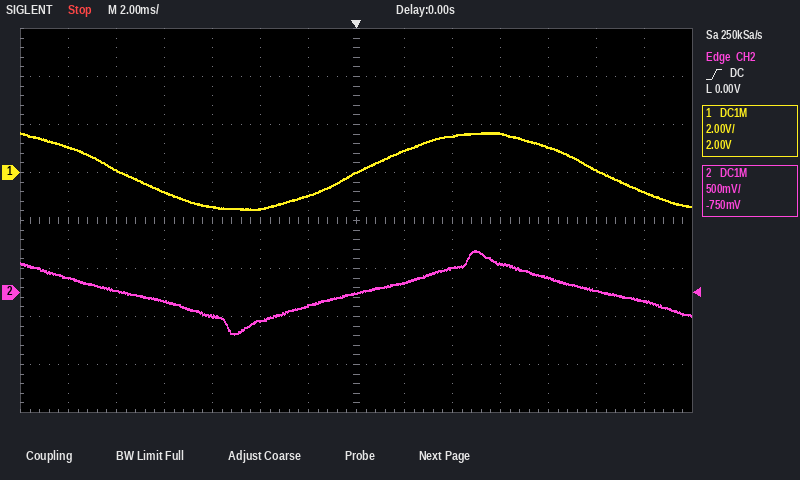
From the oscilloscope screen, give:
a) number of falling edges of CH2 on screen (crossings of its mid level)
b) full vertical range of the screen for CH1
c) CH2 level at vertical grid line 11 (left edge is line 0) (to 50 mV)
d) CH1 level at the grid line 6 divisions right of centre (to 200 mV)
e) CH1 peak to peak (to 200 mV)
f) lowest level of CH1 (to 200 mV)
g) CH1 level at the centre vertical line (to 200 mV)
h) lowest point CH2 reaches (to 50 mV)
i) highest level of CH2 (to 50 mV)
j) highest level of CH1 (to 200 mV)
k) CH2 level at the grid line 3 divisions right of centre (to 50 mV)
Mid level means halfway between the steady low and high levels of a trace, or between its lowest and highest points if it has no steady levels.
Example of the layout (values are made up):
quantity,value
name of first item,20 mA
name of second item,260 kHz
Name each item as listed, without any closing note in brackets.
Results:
quantity,value
number of falling edges of CH2 on screen,2
full vertical range of the screen for CH1,16 V
CH2 level at vertical grid line 11 (left edge is line 0),150 mV
CH1 level at the grid line 6 divisions right of centre,-800 mV
CH1 peak to peak,3.2 V
lowest level of CH1,-1.6 V
CH1 level at the centre vertical line,0.0 V
lowest point CH2 reaches,-450 mV
highest level of CH2,450 mV
highest level of CH1,1.6 V
CH2 level at the grid line 3 divisions right of centre,300 mV
